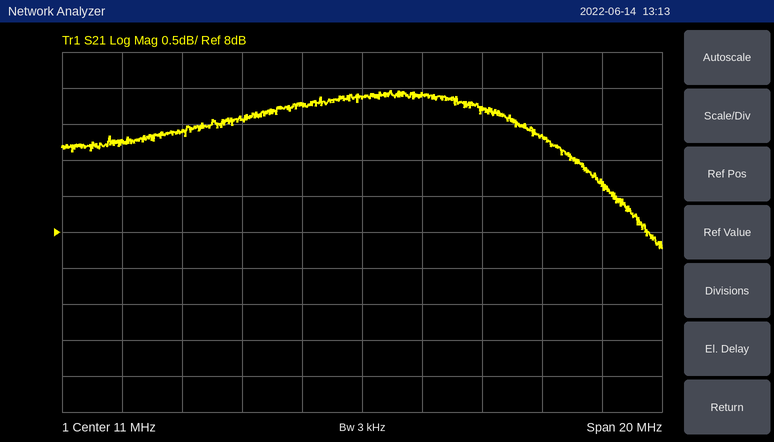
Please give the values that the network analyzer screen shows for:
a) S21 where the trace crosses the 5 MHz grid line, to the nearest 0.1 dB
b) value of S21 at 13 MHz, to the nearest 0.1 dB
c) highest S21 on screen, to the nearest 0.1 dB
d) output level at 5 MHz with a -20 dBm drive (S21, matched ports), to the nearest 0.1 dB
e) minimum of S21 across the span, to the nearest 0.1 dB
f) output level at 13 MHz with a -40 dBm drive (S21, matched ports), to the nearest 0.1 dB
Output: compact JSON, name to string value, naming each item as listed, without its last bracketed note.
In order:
{"S21 where the trace crosses the 5 MHz grid line, to the nearest 0.1 dB": "9.4 dB", "value of S21 at 13 MHz, to the nearest 0.1 dB": "9.9 dB", "highest S21 on screen, to the nearest 0.1 dB": "10.0 dB", "output level at 5 MHz with a -20 dBm drive (S21, matched ports), to the nearest 0.1 dB": "-10.6 dBm", "minimum of S21 across the span, to the nearest 0.1 dB": "7.8 dB", "output level at 13 MHz with a -40 dBm drive (S21, matched ports), to the nearest 0.1 dB": "-30.1 dBm"}
